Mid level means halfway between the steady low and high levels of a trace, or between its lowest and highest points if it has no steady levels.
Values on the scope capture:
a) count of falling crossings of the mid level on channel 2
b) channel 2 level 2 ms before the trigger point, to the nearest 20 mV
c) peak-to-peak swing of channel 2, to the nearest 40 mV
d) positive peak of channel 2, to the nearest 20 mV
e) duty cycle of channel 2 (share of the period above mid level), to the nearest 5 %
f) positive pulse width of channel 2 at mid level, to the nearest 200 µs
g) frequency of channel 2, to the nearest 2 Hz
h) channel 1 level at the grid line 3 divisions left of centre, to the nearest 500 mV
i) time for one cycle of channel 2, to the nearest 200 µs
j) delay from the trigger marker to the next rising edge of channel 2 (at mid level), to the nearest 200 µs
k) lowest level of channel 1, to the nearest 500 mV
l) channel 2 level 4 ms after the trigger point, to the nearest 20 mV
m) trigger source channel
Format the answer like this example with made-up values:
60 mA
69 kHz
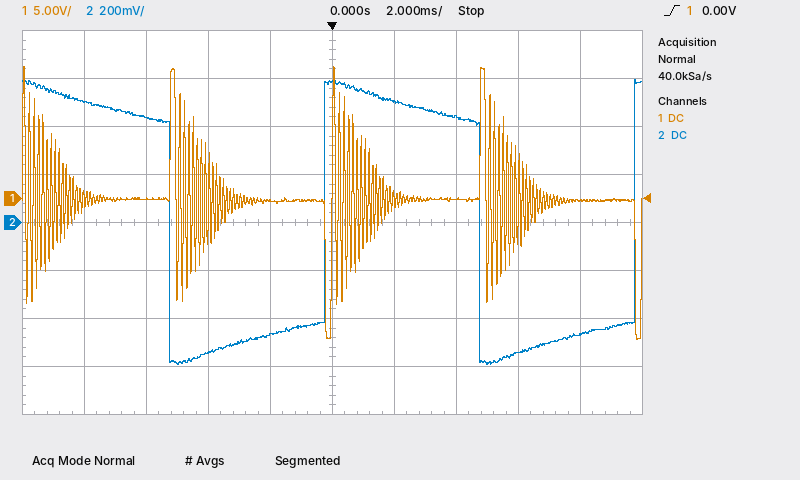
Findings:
2
-460 mV
1.20 V
600 mV
50 %
5.0 ms
100 Hz
0.0 V
10.0 ms
9.8 ms
-14.5 V
440 mV
channel 1
